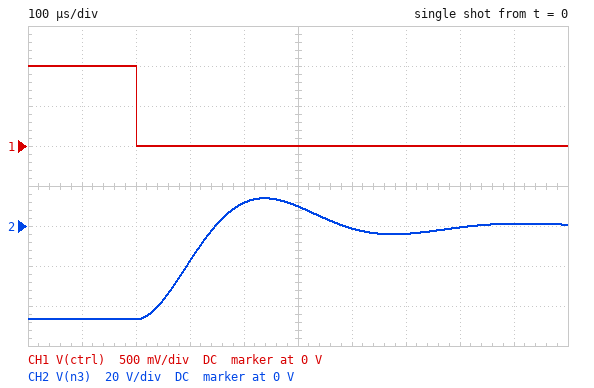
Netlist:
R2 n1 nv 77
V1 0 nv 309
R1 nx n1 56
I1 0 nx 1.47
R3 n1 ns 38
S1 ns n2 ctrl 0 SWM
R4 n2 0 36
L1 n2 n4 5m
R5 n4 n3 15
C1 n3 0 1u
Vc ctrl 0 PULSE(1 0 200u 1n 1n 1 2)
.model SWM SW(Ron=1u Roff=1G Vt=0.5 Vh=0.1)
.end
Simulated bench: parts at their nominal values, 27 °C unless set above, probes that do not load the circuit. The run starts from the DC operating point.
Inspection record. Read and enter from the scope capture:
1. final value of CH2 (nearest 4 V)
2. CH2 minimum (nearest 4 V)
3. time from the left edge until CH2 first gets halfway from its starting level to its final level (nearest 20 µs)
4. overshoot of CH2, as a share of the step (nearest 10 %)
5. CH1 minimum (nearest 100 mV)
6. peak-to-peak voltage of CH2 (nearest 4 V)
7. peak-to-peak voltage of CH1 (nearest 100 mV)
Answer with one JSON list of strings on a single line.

["0 V", "-48 V", "280 µs", "30 %", "0 V", "60 V", "1.0 V"]
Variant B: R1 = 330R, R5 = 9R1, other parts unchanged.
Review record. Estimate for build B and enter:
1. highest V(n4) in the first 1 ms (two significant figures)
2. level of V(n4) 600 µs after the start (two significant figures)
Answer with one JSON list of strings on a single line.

["16 V", "-3.4 V"]
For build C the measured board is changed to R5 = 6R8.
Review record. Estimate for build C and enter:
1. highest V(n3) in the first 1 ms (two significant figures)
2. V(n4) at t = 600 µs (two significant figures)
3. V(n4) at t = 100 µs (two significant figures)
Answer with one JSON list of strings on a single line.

["17 V", "-3.9 V", "-47 V"]
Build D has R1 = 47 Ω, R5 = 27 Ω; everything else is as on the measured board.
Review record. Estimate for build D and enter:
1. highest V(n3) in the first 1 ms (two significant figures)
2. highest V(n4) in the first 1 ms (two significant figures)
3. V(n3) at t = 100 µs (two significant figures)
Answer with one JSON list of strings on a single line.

["9.8 V", "11 V", "-47 V"]
